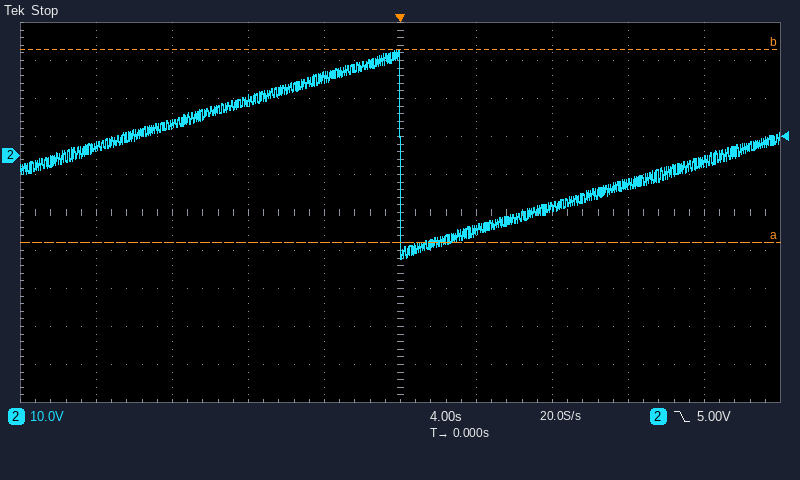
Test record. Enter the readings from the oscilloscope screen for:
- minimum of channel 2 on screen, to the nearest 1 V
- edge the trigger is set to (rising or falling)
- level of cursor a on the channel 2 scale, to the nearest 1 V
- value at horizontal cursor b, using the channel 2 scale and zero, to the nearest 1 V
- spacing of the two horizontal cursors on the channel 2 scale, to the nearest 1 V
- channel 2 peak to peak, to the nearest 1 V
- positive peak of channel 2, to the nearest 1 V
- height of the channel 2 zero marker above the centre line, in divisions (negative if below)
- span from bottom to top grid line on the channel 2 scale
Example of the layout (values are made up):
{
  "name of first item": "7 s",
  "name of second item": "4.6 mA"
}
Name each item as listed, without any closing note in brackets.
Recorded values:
{
  "minimum of channel 2 on screen, to the nearest 1 V": "-27 V",
  "edge the trigger is set to": "falling",
  "level of cursor a on the channel 2 scale, to the nearest 1 V": "-23 V",
  "value at horizontal cursor b, using the channel 2 scale and zero, to the nearest 1 V": "28 V",
  "spacing of the two horizontal cursors on the channel 2 scale, to the nearest 1 V": "51 V",
  "channel 2 peak to peak, to the nearest 1 V": "55 V",
  "positive peak of channel 2, to the nearest 1 V": "28 V",
  "height of the channel 2 zero marker above the centre line, in divisions": "+1.5 div",
  "span from bottom to top grid line on the channel 2 scale": "100 V"
}
